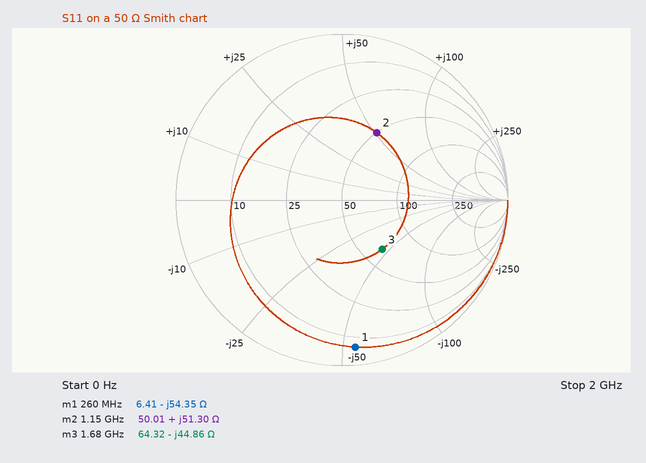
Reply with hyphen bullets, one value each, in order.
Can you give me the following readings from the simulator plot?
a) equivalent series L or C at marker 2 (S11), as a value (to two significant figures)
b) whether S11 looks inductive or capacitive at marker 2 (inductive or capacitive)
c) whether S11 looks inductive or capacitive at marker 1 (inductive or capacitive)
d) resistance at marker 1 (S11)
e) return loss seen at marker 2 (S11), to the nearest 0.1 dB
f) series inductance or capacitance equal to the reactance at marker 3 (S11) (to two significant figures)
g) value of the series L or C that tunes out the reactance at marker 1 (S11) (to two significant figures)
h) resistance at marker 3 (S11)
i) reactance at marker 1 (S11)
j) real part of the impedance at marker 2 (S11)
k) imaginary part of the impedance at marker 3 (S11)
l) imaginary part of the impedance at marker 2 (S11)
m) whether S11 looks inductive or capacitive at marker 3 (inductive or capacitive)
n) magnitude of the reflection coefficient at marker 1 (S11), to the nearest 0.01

- 7.1 nH
- inductive
- capacitive
- 6.41 Ω
- 6.8 dB
- 2.1 pF
- 33 nH
- 64.32 Ω
- -54.35 Ω
- 50.01 Ω
- -44.86 Ω
- +51.30 Ω
- capacitive
- 0.89
